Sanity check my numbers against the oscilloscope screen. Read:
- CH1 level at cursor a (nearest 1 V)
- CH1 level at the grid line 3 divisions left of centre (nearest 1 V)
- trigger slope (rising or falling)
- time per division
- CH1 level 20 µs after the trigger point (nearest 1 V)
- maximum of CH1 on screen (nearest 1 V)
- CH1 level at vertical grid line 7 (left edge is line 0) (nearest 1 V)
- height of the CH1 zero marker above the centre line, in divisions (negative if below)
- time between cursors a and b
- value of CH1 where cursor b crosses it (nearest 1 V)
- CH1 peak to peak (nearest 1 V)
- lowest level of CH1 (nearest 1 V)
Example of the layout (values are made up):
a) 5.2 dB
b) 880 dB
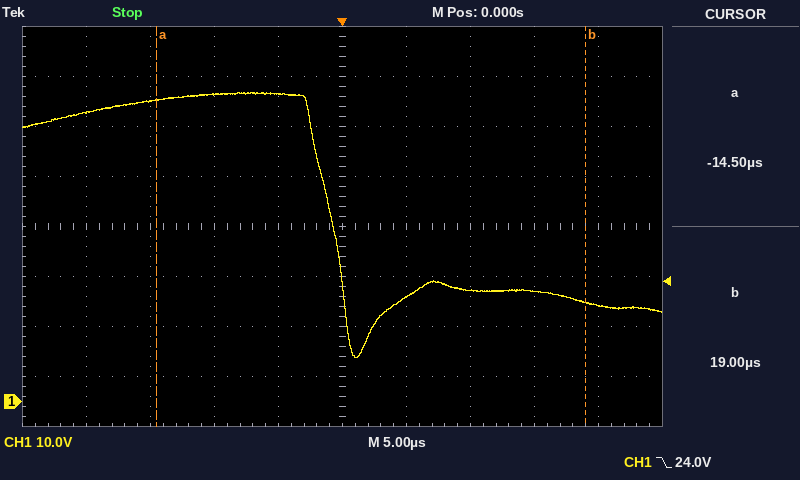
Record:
a) 60 V
b) 60 V
c) falling
d) 5 µs
e) 19 V
f) 62 V
g) 22 V
h) -3.5 div
i) 33.5 µs
j) 20 V
k) 53 V
l) 9 V
